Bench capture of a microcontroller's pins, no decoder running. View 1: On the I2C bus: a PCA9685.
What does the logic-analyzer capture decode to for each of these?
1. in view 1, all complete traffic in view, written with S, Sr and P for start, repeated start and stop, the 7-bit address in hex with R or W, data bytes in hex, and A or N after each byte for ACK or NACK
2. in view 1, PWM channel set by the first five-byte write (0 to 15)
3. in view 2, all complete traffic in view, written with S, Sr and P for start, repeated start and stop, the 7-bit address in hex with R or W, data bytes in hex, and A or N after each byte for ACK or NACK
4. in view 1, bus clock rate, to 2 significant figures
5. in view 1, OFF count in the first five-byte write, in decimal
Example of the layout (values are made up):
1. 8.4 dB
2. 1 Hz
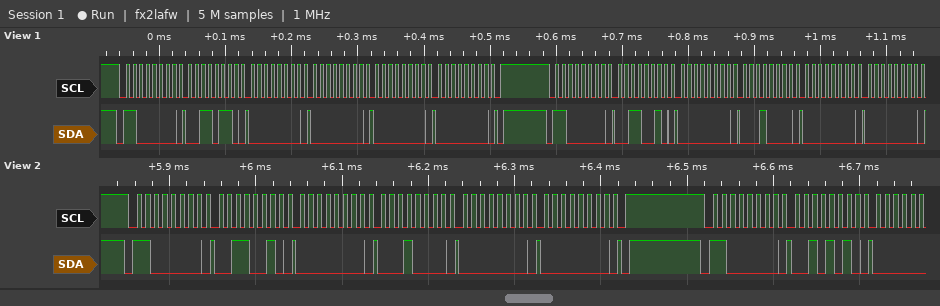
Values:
1. S 60W A 36 A 00 A 00 A 00 A 00 A P S 60W A 32 A 00 A 10 A 00 A 00 A
2. 12
3. S 60W A 32 A 00 A 10 A 00 A 00 A P S 60W A 2A A
4. 100 kHz
5. 0
